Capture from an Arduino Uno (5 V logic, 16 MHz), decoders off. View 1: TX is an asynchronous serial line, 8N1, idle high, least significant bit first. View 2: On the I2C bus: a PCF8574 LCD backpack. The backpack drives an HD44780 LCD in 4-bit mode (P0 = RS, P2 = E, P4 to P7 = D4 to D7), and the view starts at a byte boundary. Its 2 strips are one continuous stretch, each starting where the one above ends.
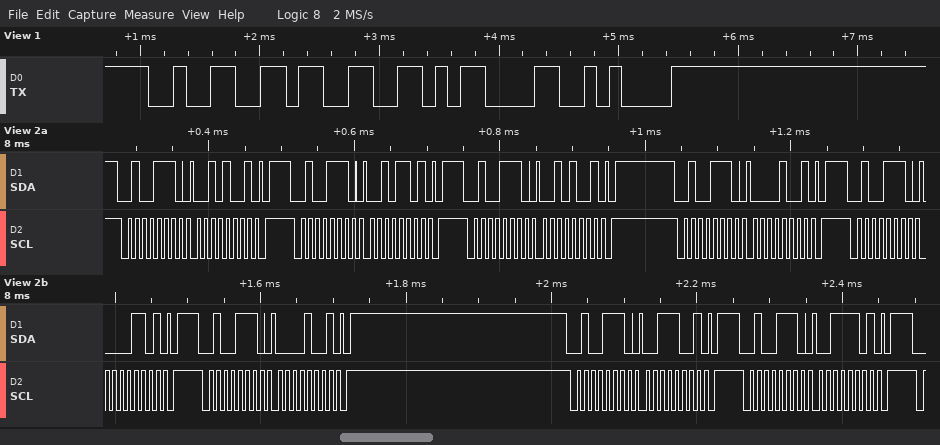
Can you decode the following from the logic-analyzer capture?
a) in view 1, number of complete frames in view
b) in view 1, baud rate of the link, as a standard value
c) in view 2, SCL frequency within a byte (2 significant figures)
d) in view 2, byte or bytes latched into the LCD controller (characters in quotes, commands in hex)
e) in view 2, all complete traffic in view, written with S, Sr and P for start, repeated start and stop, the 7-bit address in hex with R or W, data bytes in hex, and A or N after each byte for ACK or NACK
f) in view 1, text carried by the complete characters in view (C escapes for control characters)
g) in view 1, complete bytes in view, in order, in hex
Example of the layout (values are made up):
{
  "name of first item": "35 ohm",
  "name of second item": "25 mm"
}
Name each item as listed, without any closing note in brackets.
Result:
{
  "in view 1, number of complete frames in view": "4",
  "in view 1, baud rate of the link, as a standard value": "9600 baud",
  "in view 2, SCL frequency within a byte": "100 kHz",
  "in view 2, byte or bytes latched into the LCD controller": "' '",
  "in view 2, all complete traffic in view, written with S, Sr and P for start, repeated start and stop, the 7-bit address in hex with R or W, data bytes in hex, and A or N after each byte for ACK or NACK": "S 27W A 29 A P S 27W A 2D A P S 27W A 29 A P S 27W A 09 A P S 27W A 0D A P S 27W A 09 A P S 27W A 39 A P S 27W A 3D A P",
  "in view 1, text carried by the complete characters in view": "\"23\\r\\n\"",
  "in view 1, complete bytes in view, in order, in hex": "32 33 0D 0A"
}
